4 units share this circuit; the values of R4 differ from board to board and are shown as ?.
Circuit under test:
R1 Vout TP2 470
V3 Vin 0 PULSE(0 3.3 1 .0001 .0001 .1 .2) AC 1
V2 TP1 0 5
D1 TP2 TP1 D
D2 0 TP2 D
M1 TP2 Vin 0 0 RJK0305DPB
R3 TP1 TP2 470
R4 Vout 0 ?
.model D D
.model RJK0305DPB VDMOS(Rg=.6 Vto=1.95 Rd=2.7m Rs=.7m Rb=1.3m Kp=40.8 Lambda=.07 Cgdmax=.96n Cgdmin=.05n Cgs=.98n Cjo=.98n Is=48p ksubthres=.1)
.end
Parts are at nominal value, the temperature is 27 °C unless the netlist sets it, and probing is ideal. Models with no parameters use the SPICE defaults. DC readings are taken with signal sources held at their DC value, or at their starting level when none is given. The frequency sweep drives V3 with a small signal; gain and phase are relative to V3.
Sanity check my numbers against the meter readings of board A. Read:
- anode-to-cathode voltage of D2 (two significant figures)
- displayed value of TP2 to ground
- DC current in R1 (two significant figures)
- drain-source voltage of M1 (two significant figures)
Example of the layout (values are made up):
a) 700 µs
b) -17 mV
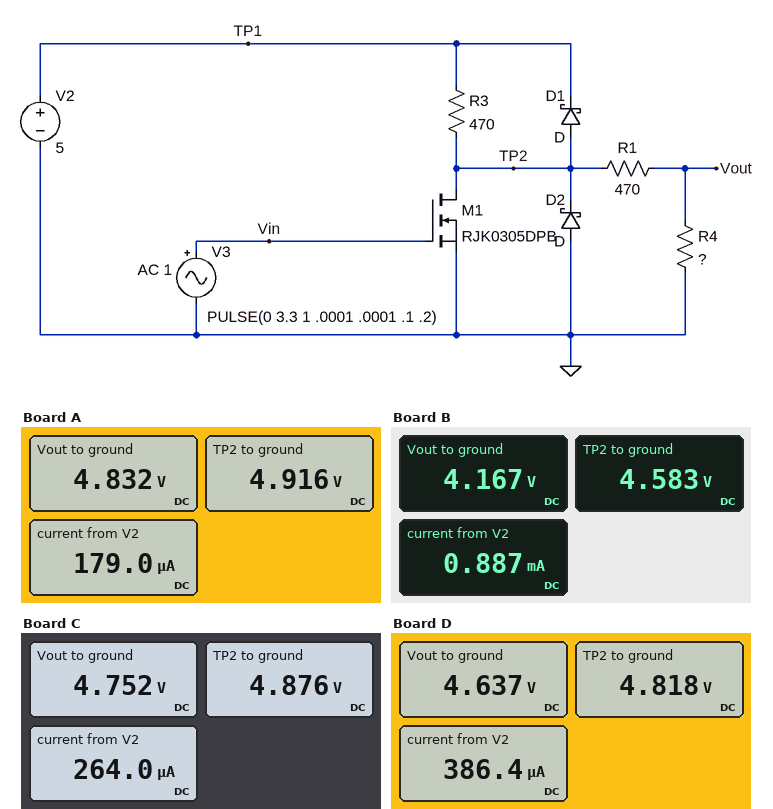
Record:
a) -4.9 V
b) 4.916 V
c) 180 µA
d) 4.9 V
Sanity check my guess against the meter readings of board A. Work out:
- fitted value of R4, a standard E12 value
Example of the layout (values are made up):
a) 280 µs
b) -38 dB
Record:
a) 27 kΩ
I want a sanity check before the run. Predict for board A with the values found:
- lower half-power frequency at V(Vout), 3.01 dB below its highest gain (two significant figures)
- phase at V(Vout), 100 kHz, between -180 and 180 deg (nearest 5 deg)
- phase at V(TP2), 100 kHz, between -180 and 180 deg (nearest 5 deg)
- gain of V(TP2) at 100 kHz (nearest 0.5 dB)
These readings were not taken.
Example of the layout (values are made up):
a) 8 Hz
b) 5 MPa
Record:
a) 700 kHz
b) 80 deg
c) 80 deg
d) -29.0 dB
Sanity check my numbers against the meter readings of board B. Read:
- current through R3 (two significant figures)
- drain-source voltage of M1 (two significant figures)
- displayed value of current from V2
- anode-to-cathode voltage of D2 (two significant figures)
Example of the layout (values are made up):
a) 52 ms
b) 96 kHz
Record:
a) 890 µA
b) 4.6 V
c) 0.887 mA
d) -4.6 V
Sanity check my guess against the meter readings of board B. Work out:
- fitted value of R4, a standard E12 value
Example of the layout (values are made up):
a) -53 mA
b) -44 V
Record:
a) 4.7 kΩ
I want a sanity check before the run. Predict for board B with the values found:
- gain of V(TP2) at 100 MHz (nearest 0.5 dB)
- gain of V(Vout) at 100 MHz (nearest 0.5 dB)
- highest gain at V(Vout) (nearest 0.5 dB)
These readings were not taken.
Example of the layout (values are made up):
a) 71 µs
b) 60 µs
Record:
a) -12.5 dB
b) -13.5 dB
c) -13.0 dB
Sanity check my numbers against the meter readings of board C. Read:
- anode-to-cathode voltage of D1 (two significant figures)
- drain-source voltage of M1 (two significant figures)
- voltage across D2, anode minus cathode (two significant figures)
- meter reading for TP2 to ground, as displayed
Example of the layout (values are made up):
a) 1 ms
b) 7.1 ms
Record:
a) -120 mV
b) 4.9 V
c) -4.9 V
d) 4.876 V
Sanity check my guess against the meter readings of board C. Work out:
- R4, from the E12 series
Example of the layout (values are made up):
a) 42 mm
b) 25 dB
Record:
a) 18 kΩ
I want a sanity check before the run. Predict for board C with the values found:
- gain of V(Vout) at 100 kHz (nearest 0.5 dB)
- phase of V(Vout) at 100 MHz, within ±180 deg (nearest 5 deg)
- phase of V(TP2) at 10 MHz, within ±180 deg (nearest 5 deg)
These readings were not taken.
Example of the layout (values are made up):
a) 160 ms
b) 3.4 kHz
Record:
a) -29.5 dB
b) -20 deg
c) 0 deg
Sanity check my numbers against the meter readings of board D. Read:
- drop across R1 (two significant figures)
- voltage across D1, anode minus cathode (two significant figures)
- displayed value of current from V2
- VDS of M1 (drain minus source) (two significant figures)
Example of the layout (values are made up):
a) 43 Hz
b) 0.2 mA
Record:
a) 180 mV
b) -180 mV
c) 386.4 µA
d) 4.8 V
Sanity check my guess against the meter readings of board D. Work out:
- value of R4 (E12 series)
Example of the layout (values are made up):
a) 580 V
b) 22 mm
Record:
a) 12 kΩ
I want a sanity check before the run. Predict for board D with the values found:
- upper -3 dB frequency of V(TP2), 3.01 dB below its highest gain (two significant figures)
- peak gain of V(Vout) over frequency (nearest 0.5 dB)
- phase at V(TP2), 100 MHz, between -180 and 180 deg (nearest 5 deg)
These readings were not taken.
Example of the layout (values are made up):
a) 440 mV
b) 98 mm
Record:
a) 250 MHz
b) -12.5 dB
c) -20 deg
